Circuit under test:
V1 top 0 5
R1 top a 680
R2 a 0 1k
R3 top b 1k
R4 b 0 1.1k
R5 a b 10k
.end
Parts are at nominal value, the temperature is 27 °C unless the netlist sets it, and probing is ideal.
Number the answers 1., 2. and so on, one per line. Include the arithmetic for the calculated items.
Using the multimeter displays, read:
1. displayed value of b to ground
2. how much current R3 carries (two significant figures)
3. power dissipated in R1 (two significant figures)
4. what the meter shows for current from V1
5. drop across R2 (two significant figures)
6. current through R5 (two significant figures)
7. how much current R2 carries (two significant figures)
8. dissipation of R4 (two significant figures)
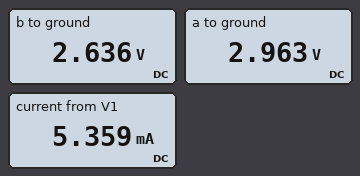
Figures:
1. 2.636 V
2. (5 V - 2.636 V) / 1 kΩ = 2.4 mA
3. (5 V - 2.963 V)^2 / 680 Ω = 6.1 mW
4. 5.359 mA
5. 2.963 V = 3.0 V
6. (2.963 V - 2.636 V) / 10 kΩ = 33 µA
7. (2.963 V) / 1 kΩ = 3.0 mA
8. (2.636 V)^2 / 1.1 kΩ = 6.3 mW
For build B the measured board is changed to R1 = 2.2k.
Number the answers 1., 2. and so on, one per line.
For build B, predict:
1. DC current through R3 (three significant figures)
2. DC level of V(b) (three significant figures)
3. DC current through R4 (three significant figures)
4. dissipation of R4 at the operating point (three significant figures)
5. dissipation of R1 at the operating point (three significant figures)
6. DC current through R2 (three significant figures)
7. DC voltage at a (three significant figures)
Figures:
1. 2.43 mA
2. 2.57 V
3. 2.34 mA
4. 6.00 mW
5. 5.17 mW
6. 1.63 mA
7. 1.63 V
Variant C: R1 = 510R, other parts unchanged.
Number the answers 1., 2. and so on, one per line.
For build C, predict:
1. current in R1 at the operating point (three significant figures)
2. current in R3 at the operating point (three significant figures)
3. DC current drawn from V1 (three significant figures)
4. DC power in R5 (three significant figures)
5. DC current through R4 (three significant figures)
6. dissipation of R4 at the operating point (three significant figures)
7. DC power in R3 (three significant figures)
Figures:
1. 3.35 mA
2. 2.35 mA
3. 5.70 mA
4. 40.6 µW
5. 2.41 mA
6. 6.40 mW
7. 5.51 mW
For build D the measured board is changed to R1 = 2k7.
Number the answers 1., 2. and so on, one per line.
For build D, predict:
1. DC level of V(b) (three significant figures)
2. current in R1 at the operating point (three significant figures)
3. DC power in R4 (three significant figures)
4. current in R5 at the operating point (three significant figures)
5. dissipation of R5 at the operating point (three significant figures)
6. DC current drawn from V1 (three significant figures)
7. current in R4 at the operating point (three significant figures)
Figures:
1. 2.56 V
2. 1.32 mA
3. 5.96 mW
4. 113 µA
5. 127 µW
6. 3.76 mA
7. 2.33 mA
